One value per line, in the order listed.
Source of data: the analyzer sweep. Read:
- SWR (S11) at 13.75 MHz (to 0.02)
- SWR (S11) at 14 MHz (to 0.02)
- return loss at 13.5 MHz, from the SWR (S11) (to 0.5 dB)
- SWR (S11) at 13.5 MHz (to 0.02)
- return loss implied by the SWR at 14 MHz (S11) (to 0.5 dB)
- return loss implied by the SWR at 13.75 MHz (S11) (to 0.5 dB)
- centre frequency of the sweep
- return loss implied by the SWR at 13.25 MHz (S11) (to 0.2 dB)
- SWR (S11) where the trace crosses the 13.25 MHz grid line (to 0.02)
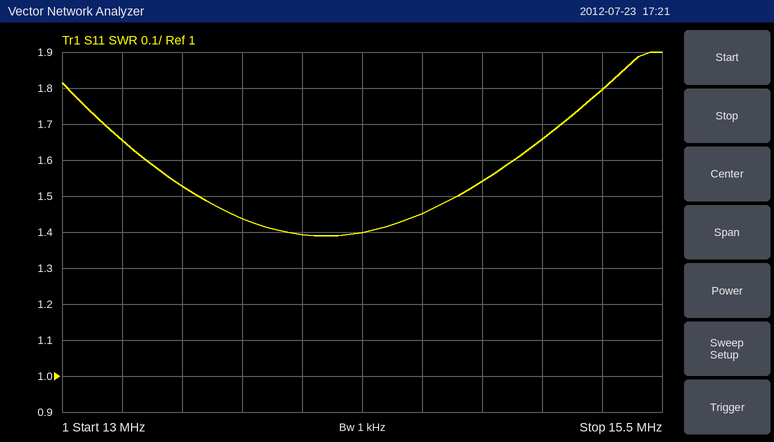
1.44
1.40
13.5 dB
1.52
15.5 dB
15.0 dB
14.25 MHz
12.2 dB
1.66
